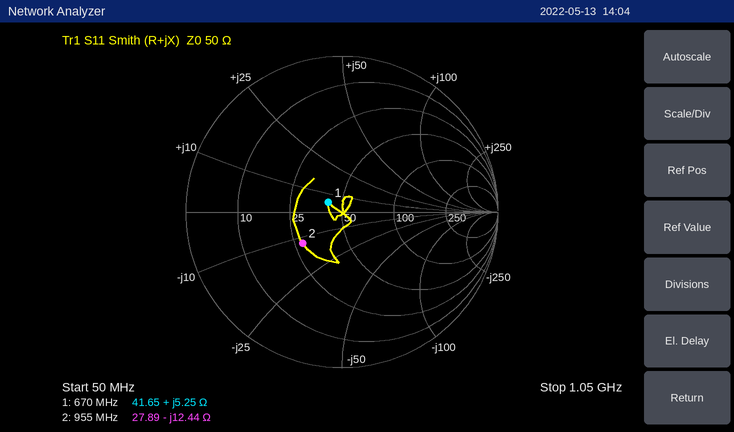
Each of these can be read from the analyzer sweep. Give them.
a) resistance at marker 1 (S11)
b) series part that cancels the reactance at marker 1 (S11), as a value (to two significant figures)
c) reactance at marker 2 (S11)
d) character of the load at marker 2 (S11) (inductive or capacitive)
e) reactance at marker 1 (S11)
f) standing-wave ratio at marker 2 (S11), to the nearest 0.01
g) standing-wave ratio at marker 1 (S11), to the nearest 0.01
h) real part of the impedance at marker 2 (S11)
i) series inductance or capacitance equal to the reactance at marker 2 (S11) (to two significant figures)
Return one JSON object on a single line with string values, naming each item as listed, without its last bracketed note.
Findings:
{"resistance at marker 1": "41.65 Ω", "series part that cancels the reactance at marker 1 (S11), as a value": "45 pF", "reactance at marker 2": "-12.44 Ω", "character of the load at marker 2 (S11)": "capacitive", "reactance at marker 1": "+5.25 Ω", "standing-wave ratio at marker 2 (S11), to the nearest 0.01": "1.95", "standing-wave ratio at marker 1 (S11), to the nearest 0.01": "1.24", "real part of the impedance at marker 2": "27.89 Ω", "series inductance or capacitance equal to the reactance at marker 2 (S11)": "13 pF"}
